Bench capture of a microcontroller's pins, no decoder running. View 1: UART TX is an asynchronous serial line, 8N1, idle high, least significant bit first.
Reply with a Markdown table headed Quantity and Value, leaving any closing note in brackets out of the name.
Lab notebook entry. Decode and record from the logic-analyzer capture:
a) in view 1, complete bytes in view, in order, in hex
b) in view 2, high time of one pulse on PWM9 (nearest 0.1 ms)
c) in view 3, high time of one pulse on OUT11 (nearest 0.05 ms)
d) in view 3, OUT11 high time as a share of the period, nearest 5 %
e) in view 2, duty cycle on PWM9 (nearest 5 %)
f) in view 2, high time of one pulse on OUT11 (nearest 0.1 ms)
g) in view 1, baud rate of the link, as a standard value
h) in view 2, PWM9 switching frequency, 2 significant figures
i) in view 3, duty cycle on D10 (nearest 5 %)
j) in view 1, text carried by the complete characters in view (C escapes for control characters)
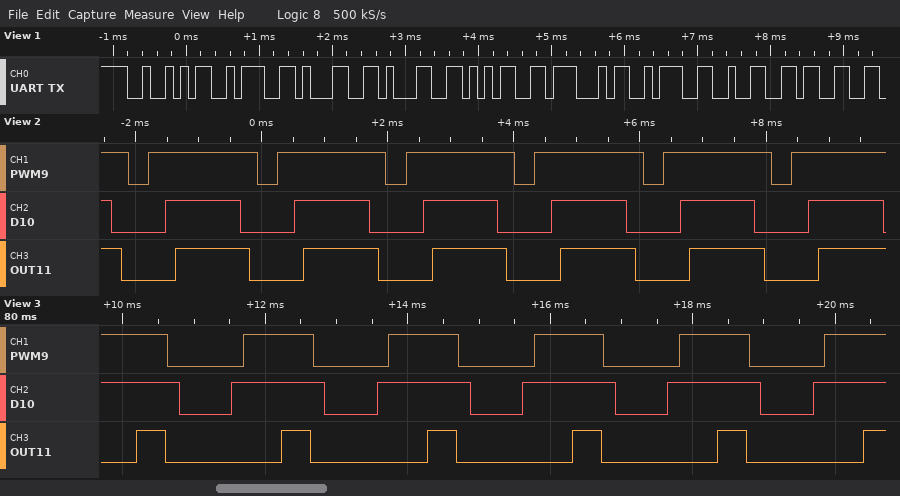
| Quantity | Value |
|---|---|
| in view 1, complete bytes in view, in order, in hex | 52 3A 31 31 35 47 3A 32 33 |
| in view 2, high time of one pulse on PWM9 | 1.7 ms |
| in view 3, high time of one pulse on OUT11 | 0.40 ms |
| in view 3, OUT11 high time as a share of the period, nearest 5 % | 20 % |
| in view 2, duty cycle on PWM9 | 85 % |
| in view 2, high time of one pulse on OUT11 | 1.2 ms |
| in view 1, baud rate of the link, as a standard value | 9600 baud |
| in view 2, PWM9 switching frequency, 2 significant figures | 490 Hz |
| in view 3, duty cycle on D10 | 65 % |
| in view 1, text carried by the complete characters in view | "R:115G:23" |
